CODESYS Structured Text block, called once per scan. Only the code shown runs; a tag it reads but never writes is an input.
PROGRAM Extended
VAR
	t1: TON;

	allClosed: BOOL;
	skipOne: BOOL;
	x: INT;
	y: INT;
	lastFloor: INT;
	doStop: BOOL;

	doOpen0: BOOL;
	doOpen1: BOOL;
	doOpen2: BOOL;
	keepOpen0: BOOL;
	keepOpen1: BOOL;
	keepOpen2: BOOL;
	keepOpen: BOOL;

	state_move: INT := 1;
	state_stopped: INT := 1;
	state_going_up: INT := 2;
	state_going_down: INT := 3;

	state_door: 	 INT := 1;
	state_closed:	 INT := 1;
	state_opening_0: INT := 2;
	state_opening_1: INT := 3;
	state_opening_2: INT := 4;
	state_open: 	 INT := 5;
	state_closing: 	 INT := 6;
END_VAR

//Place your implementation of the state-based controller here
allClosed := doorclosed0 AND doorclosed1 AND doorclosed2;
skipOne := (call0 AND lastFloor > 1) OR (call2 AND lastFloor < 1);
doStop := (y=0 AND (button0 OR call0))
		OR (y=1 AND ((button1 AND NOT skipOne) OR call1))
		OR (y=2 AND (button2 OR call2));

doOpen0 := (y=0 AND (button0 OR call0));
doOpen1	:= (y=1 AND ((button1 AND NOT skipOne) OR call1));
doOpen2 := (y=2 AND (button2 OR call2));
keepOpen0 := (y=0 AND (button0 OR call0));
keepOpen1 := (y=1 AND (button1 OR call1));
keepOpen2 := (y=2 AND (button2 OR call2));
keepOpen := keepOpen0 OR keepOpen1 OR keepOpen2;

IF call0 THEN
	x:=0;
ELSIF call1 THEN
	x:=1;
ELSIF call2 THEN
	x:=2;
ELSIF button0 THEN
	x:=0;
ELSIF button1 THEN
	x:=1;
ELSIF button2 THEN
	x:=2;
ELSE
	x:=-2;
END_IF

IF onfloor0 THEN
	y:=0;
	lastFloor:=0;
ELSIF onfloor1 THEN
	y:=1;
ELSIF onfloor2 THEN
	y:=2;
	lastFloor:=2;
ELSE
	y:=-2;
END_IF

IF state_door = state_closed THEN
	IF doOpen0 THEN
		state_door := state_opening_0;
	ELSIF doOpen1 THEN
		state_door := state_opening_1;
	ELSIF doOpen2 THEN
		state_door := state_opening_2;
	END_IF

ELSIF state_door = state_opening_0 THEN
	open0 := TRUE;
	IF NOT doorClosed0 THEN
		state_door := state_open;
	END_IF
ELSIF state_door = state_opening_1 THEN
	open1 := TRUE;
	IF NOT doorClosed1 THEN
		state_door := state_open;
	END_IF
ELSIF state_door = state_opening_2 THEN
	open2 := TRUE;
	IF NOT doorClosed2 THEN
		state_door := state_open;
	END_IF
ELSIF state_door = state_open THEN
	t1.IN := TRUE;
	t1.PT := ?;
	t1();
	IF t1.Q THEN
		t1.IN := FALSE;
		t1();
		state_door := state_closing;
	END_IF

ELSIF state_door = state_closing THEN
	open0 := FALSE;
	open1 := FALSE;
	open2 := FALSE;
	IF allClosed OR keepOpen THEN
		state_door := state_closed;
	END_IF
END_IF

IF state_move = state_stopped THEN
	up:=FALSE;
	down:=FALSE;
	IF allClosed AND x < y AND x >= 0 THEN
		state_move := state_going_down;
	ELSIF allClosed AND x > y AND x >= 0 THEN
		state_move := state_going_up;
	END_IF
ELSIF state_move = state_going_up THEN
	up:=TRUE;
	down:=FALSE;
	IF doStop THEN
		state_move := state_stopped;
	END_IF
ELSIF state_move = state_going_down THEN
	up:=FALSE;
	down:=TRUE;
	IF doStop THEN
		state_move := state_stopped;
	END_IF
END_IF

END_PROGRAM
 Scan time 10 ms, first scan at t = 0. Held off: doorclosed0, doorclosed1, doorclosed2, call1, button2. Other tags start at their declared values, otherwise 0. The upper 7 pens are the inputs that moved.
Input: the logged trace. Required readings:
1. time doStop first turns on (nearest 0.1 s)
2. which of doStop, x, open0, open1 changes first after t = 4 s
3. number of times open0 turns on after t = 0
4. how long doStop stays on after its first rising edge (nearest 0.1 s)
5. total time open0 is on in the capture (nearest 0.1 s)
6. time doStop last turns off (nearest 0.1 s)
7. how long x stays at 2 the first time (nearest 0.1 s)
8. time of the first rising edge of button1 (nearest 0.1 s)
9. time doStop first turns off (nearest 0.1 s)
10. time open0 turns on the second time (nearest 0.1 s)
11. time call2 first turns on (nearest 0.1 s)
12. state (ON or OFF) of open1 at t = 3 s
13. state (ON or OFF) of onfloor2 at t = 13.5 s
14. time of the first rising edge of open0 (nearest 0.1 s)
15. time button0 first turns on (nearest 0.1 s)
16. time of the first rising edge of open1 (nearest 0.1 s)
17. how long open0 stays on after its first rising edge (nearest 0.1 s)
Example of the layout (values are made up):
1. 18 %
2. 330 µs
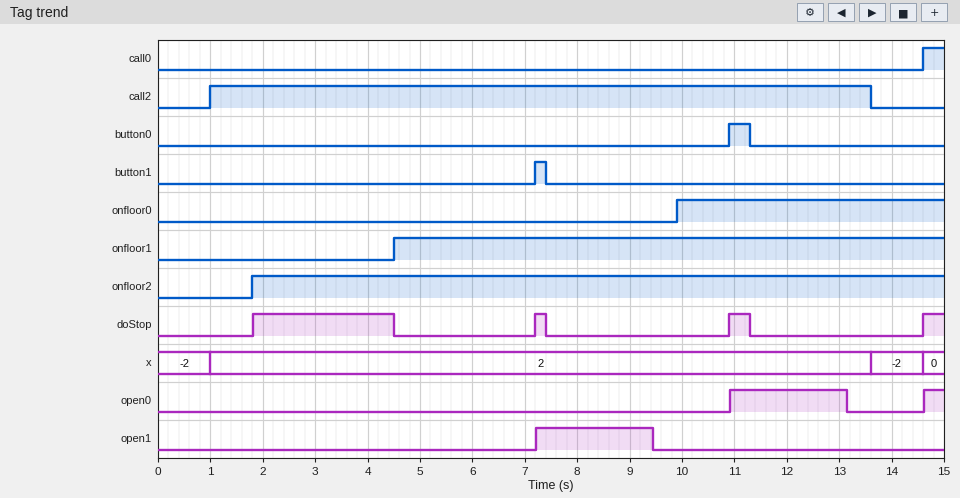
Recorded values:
1. 1.8 s
2. doStop
3. 2
4. 2.7 s
5. 2.6 s
6. 11.3 s
7. 12.6 s
8. 7.2 s
9. 4.5 s
10. 14.6 s
11. 1.0 s
12. OFF
13. ON
14. 10.9 s
15. 10.9 s
16. 7.2 s
17. 2.2 s
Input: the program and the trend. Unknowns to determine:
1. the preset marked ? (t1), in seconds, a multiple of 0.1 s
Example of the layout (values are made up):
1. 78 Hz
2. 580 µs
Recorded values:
1. 2.2 s
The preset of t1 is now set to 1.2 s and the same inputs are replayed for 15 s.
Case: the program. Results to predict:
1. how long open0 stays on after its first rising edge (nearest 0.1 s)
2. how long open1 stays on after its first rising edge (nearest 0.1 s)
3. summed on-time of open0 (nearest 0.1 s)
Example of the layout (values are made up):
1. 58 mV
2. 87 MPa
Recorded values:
1. 1.2 s
2. 1.2 s
3. 1.6 s
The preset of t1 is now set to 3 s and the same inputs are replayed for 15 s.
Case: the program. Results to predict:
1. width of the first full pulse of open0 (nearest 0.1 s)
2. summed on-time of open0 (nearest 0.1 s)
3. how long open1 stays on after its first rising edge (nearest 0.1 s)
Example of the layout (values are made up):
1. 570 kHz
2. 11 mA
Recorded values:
1. 3.0 s
2. 3.4 s
3. 3.0 s
